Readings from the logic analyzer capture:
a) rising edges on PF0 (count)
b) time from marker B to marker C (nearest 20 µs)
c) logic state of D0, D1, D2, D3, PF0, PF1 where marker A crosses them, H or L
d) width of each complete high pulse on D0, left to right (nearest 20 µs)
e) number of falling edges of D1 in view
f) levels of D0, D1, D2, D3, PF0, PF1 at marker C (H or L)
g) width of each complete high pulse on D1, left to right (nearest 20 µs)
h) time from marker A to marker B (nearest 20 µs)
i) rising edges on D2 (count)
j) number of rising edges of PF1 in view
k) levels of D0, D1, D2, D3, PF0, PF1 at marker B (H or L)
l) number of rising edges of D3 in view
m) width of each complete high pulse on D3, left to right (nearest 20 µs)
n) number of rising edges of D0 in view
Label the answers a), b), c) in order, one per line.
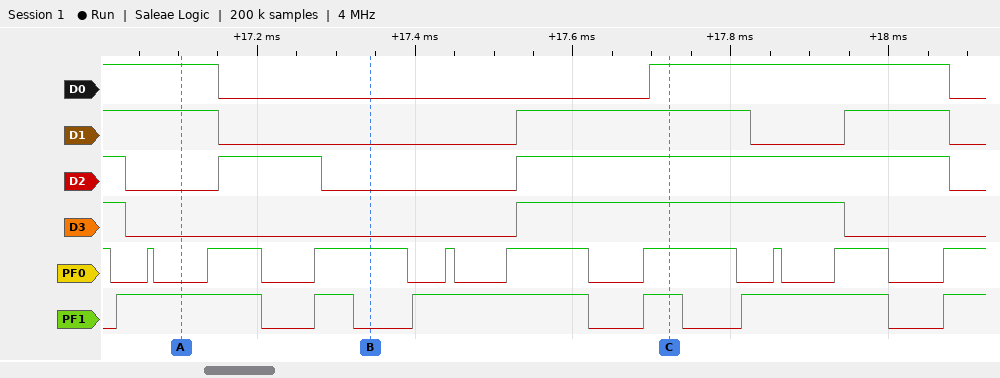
a) 9
b) 380 µs
c) D0=H, D1=H, D2=L, D3=L, PF0=L, PF1=H
d) 380 µs
e) 3
f) D0=H, D1=H, D2=H, D3=H, PF0=H, PF1=H
g) 300 µs, 140 µs
h) 240 µs
i) 2
j) 6
k) D0=L, D1=L, D2=L, D3=L, PF0=H, PF1=L
l) 1
m) 420 µs
n) 1
